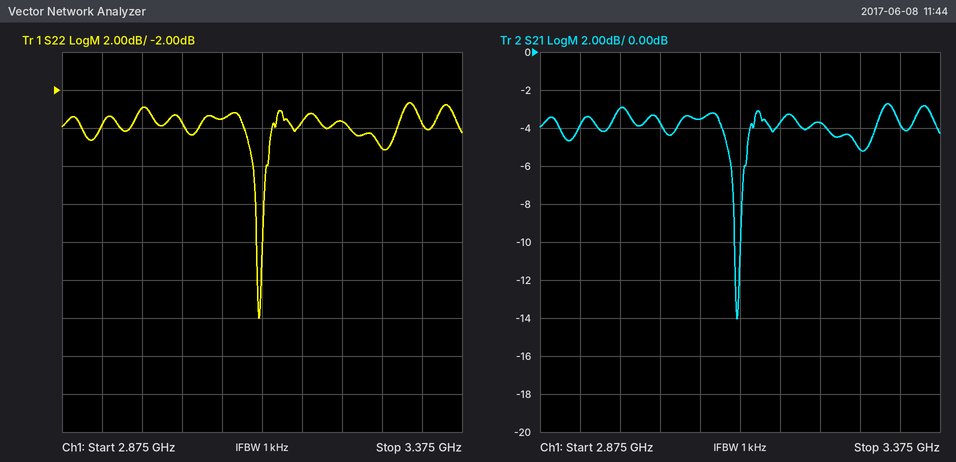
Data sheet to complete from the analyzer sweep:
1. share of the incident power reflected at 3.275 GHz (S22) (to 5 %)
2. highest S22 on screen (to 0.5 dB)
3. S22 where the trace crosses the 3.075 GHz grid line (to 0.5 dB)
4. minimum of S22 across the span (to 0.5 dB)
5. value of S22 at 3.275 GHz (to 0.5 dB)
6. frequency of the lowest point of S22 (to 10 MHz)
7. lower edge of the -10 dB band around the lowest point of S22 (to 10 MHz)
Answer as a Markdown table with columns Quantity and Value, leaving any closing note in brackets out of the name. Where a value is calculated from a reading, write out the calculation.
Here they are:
| Quantity | Value |
|---|---|
| share of the incident power reflected at 3.275 GHz (S22) | 10^(-5/10) ≈ 31.6 %, so 30 % to the nearest 5 % |
| highest S22 on screen | -2.5 dB |
| S22 where the trace crosses the 3.075 GHz grid line | -3.5 dB |
| minimum of S22 across the span | -14.0 dB |
| value of S22 at 3.275 GHz | -5.0 dB |
| frequency of the lowest point of S22 | 3.12 GHz |
| lower edge of the -10 dB band around the lowest point of S22 | 3.12 GHz |
